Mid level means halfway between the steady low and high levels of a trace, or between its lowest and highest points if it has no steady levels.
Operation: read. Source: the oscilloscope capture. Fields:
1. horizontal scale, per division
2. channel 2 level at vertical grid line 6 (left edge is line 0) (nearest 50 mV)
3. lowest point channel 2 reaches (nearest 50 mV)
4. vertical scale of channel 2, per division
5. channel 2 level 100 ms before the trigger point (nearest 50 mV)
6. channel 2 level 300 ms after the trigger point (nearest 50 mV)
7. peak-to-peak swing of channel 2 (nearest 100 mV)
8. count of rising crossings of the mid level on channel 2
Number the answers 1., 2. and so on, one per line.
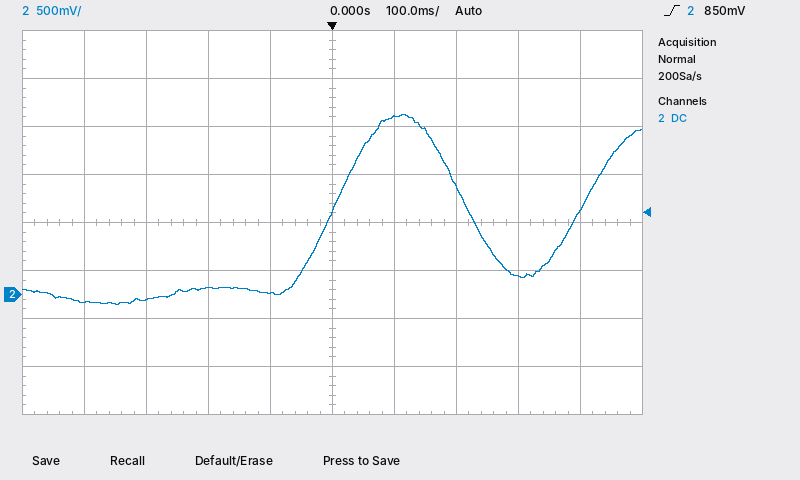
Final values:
1. 100 ms
2. 1.85 V
3. -100 mV
4. 500 mV
5. 0 mV
6. 200 mV
7. 2.00 V
8. 2
